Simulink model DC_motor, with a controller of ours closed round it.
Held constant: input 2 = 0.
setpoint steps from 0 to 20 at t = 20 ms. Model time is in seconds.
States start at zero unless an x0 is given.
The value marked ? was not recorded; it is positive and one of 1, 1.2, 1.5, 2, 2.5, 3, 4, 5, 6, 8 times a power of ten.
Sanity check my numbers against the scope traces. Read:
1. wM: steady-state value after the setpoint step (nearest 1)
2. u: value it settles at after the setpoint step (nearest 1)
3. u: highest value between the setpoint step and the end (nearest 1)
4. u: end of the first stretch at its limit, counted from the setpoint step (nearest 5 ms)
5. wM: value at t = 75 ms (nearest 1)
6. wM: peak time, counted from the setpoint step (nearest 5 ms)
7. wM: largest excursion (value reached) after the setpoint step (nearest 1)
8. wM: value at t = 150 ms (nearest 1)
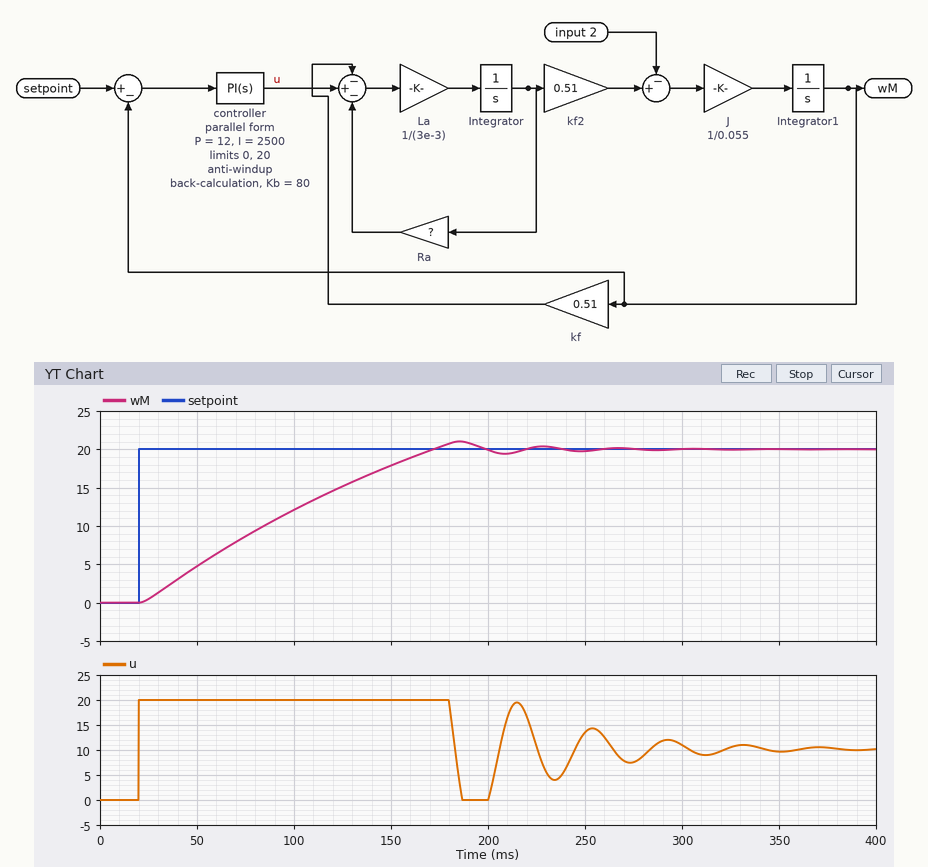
20
10
20
160 ms
9
165 ms
21
18
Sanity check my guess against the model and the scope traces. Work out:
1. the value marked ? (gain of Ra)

1
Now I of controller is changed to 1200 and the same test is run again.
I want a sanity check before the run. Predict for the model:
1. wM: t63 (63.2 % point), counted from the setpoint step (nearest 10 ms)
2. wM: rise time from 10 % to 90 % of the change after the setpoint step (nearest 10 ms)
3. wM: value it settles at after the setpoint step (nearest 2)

80 ms
120 ms
20
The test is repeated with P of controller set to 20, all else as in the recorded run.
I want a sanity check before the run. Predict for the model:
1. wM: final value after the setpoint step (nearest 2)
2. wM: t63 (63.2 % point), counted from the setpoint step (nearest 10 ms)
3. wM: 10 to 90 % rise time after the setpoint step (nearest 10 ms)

20
80 ms
120 ms
